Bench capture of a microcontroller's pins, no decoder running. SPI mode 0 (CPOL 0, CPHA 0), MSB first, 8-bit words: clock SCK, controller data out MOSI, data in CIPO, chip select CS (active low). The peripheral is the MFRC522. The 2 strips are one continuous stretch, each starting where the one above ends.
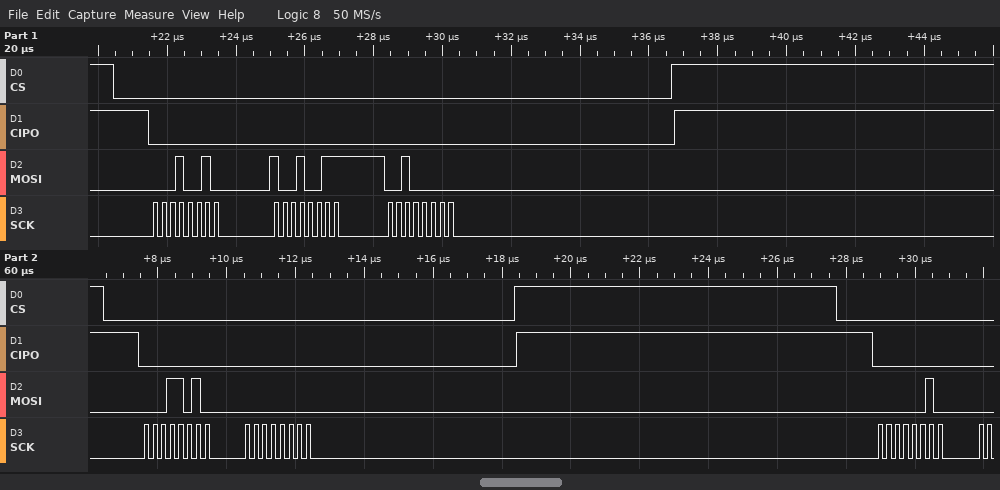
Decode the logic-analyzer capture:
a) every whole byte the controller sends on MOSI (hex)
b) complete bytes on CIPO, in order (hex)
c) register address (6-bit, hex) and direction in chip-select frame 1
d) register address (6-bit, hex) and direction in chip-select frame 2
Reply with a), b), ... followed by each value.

a) 12 93 20 1A 00 02
b) 00 00 00 00 00 00
c) 0x09 write
d) 0x0D write
